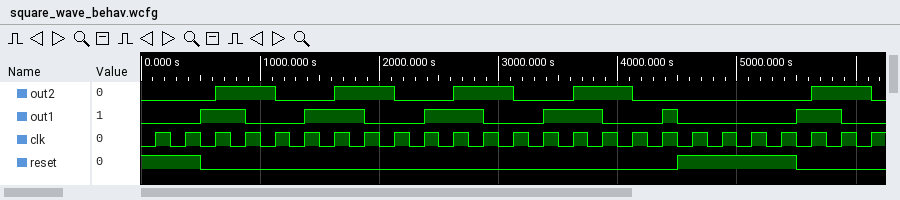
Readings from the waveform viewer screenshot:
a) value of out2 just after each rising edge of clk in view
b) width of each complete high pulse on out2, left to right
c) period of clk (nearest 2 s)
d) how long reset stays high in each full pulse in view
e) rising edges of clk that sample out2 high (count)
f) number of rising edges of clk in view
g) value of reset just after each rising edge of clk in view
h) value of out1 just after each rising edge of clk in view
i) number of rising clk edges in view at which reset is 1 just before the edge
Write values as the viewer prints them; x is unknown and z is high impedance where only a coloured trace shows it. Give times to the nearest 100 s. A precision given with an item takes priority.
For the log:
0 0 1 1 0 0 1 1 0 0 1 1 0 0 1 1 0 0 0 0 0 0 1 1 0
500 s, 500 s, 500 s, 500 s, 500 s
250 s
1000 s
10
25
1 1 0 0 0 0 0 0 0 0 0 0 0 0 0 0 0 0 1 1 1 1 0 0 0
0 0 1 0 0 1 1 0 0 1 1 0 0 1 1 0 0 1 0 0 0 0 1 0 0
6
